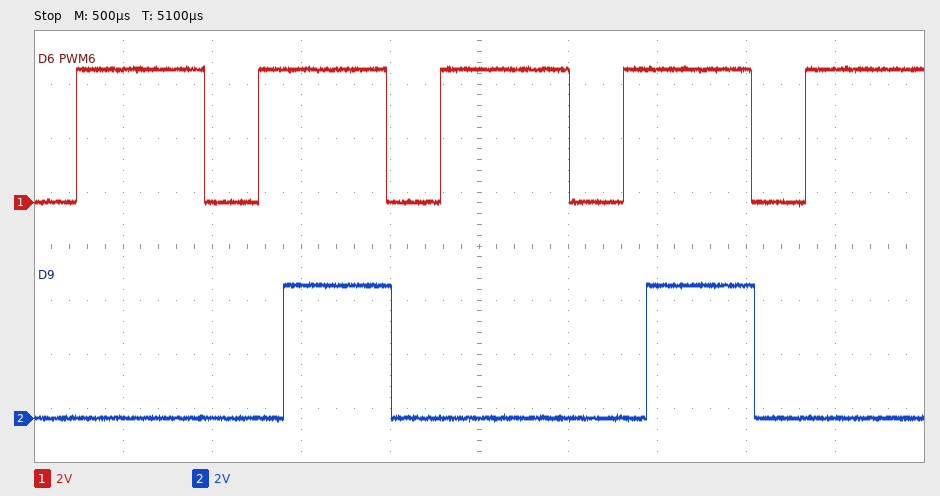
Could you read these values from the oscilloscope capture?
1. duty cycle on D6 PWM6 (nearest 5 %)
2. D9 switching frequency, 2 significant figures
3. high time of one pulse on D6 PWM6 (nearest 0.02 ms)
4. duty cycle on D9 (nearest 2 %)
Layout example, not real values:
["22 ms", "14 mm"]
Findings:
["70 %", "490 Hz", "0.72 ms", "30 %"]
